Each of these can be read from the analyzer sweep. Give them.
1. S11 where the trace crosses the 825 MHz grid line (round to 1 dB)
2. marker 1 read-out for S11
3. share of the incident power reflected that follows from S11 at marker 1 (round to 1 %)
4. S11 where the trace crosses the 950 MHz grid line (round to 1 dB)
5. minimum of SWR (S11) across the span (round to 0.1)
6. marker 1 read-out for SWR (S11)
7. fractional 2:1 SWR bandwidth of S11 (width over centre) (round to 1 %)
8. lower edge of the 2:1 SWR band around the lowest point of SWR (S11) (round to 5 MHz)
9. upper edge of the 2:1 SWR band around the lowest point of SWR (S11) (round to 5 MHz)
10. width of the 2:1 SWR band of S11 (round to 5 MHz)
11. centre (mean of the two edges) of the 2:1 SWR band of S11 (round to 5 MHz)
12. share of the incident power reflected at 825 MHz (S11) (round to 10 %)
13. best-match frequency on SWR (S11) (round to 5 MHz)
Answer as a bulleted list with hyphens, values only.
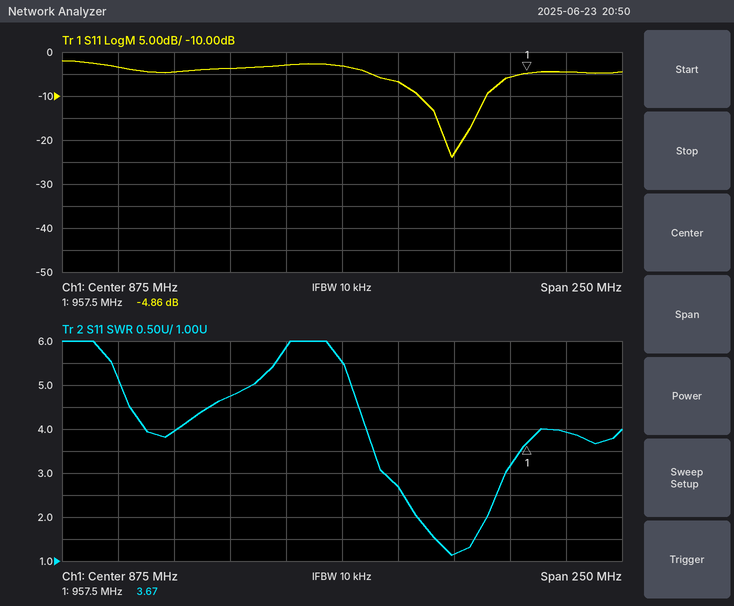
- -4 dB
- -4.86 dB
- 33 %
- -6 dB
- 1.1
- 3.67
- 3 %
- 910 MHz
- 940 MHz
- 30 MHz
- 925 MHz
- 40 %
- 925 MHz
